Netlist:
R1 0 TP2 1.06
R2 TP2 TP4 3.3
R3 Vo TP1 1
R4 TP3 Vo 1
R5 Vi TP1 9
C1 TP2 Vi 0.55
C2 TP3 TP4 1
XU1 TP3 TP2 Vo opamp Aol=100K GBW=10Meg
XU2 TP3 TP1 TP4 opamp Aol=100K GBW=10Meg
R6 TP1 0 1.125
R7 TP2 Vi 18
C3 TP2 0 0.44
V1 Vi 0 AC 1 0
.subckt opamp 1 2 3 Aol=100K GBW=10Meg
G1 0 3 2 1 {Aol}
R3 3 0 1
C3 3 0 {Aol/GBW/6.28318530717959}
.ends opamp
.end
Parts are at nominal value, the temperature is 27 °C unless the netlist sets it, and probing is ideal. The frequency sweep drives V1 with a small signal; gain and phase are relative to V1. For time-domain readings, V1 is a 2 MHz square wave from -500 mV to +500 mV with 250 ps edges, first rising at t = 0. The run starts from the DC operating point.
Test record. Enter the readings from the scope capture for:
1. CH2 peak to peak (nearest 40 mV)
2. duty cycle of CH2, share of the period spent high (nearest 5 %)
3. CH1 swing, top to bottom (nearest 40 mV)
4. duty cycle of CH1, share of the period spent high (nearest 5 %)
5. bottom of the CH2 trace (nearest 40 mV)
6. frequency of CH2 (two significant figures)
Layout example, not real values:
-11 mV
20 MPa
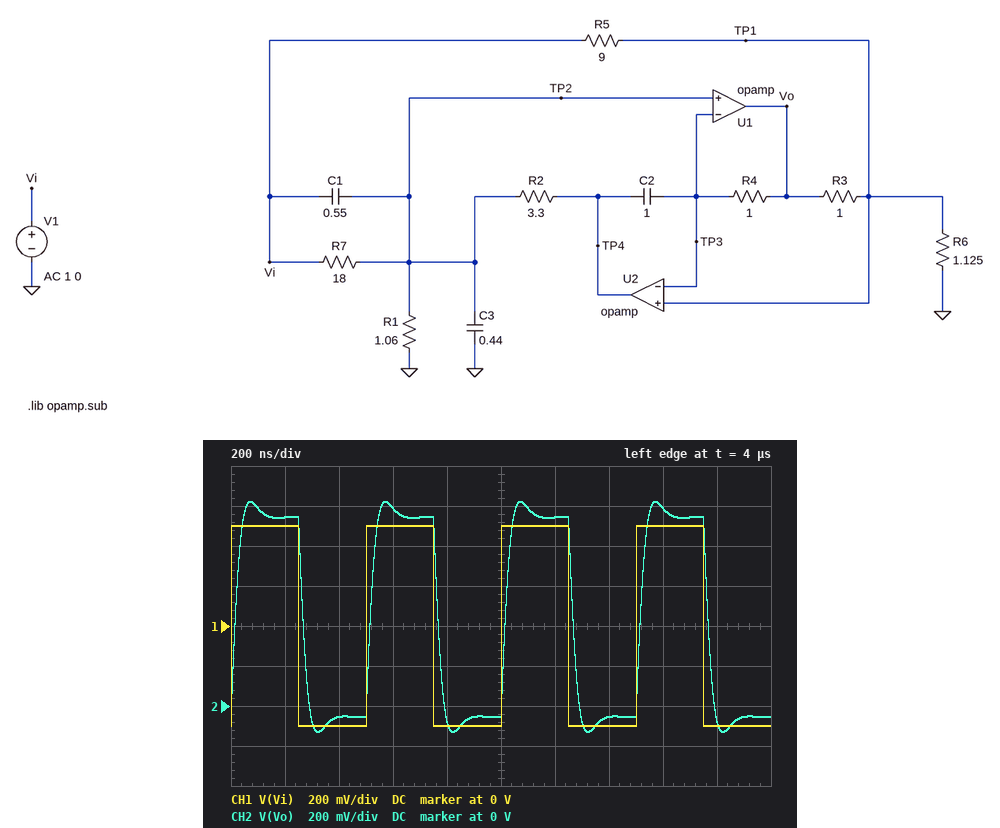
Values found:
1.16 V
50 %
1.00 V
50 %
-120 mV
2.0 MHz
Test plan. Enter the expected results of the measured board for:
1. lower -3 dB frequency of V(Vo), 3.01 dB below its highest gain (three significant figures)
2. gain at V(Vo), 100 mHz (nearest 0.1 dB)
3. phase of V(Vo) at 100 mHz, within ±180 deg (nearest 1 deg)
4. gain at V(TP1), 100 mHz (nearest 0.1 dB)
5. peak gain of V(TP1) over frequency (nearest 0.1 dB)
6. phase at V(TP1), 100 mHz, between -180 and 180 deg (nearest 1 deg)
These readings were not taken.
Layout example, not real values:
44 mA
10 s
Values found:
131 mHz
-5.0 dB
82 deg
-10.6 dB
-5.1 dB
71 deg
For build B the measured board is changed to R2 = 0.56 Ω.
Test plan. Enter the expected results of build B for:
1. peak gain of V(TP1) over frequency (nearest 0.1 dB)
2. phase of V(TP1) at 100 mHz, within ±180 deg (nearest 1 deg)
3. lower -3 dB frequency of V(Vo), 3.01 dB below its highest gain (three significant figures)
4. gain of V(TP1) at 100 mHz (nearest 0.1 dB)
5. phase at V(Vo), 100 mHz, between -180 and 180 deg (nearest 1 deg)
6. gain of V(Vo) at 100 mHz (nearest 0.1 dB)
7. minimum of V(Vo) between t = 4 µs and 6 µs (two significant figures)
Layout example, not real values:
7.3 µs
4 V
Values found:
-3.2 dB
94 deg
187 mHz
-31.7 dB
156 deg
-18.0 dB
-130 mV
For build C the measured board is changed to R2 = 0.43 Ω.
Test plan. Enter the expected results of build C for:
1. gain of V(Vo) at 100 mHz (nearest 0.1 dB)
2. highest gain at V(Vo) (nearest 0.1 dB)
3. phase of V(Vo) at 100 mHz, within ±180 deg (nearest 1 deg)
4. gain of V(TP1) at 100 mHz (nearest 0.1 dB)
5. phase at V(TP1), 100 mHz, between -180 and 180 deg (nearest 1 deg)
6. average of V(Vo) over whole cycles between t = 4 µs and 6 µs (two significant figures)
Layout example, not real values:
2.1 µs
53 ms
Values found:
-23.7 dB
3.4 dB
162 deg
-31.5 dB
22 deg
440 mV
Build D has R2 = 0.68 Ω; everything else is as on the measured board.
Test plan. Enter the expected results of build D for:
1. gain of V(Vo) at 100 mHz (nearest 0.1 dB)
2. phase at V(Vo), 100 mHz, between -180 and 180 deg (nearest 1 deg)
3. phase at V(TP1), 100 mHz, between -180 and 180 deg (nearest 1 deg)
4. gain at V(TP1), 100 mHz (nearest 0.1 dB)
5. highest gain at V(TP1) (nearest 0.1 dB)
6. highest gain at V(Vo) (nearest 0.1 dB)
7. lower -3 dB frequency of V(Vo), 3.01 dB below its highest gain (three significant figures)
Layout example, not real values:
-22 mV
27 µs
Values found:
-14.8 dB
150 deg
117 deg
-25.8 dB
-3.7 dB
1.8 dB
171 mHz
